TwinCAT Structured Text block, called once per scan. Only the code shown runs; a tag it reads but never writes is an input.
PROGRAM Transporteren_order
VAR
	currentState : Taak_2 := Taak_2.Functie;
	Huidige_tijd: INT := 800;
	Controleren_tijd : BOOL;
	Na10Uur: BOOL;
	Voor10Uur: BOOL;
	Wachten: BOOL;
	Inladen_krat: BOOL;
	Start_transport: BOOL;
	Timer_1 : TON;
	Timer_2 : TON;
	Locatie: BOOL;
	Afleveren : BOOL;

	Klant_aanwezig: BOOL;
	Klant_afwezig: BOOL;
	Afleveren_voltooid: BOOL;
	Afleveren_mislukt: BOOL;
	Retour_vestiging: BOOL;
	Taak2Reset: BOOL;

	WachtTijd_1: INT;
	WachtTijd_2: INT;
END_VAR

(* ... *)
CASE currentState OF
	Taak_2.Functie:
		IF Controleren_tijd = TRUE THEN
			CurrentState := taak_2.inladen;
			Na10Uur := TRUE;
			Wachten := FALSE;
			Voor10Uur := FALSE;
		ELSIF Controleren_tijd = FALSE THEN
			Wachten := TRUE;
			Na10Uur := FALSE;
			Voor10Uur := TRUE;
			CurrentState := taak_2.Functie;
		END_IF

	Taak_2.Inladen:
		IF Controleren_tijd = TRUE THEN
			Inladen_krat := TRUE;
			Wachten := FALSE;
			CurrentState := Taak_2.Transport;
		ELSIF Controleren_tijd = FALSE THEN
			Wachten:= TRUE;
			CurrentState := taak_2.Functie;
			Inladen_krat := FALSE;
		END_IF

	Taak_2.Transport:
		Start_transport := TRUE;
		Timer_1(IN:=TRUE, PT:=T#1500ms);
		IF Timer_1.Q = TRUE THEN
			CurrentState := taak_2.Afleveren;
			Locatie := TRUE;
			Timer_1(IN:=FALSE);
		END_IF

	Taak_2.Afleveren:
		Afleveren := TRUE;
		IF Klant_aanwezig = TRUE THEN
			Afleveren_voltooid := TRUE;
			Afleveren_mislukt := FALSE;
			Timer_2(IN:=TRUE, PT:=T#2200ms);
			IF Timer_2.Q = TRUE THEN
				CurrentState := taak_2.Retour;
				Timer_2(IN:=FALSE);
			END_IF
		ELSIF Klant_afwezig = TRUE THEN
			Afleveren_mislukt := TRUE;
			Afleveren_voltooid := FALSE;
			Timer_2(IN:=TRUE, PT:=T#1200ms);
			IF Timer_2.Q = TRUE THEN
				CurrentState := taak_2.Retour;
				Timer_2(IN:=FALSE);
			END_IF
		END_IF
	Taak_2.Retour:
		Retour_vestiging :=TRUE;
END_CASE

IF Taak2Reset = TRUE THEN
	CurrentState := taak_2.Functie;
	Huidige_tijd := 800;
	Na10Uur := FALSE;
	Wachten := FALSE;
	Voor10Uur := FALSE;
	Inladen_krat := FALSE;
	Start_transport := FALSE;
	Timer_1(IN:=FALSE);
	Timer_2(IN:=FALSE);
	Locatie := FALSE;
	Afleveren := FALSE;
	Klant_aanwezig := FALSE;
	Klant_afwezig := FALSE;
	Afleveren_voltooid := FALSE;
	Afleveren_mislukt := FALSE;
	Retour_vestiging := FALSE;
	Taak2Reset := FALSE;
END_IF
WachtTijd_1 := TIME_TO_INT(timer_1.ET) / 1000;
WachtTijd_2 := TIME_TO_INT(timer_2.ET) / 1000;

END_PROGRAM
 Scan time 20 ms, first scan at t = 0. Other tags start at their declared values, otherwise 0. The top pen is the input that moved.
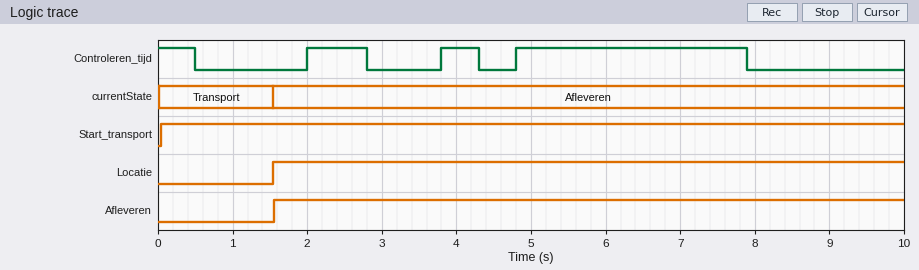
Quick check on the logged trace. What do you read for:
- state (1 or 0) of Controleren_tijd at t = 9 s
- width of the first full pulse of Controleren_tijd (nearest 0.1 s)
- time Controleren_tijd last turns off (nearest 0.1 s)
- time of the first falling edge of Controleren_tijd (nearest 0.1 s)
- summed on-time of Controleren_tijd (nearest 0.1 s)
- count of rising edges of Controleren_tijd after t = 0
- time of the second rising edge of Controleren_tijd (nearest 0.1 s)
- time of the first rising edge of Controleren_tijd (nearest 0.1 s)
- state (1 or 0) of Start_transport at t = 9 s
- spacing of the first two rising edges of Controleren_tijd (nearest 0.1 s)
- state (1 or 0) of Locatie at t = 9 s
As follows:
0
0.8 s
7.9 s
0.5 s
4.9 s
3
3.8 s
2.0 s
1
1.8 s
1
